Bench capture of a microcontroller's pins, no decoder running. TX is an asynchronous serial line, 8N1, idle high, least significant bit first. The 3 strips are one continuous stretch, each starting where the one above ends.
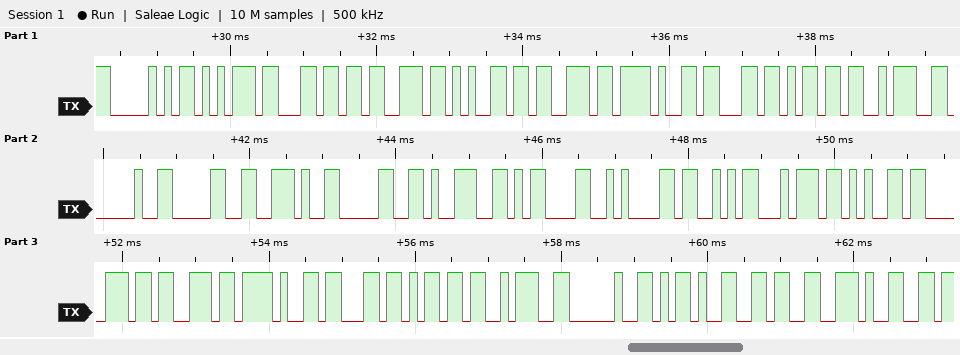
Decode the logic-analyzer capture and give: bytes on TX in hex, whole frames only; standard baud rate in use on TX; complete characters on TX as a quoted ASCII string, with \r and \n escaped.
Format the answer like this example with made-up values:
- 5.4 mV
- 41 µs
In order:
- 50 75 6C 73 65 73 2F 63 6D 3A 20 30 2E 30 39 0D 0A 53 74 65 70 73 2F 63 6D 3A 20 2D 36 2E
- 9600 baud
- "Pulses/cm: 0.09\r\nSteps/cm: -6."
